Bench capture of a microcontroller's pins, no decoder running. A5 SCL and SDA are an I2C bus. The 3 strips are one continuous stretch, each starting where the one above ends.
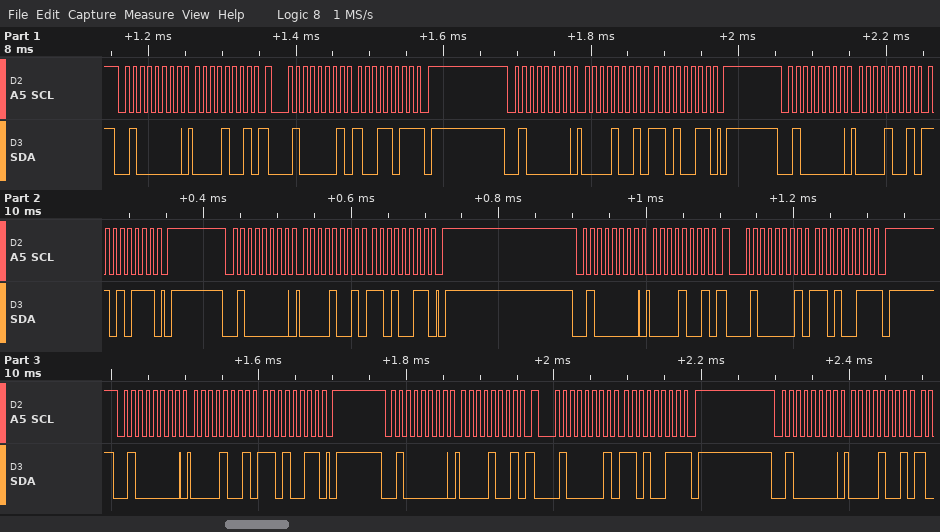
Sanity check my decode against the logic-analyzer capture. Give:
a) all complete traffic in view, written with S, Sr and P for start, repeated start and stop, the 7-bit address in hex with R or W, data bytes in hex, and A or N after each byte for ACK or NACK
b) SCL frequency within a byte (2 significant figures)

S 20W A 09 A Sr 20R A 9B N P S 20W A 09 A D3 A P S 20W A 09 A D7 A P S 20W A 09 A D3 A P S 20W A 09 A Sr 20R A D3 N P S 20W A 09 A D3 A P S 20W A 09 A Sr 20R A D3 N P S 20W A 09 A
100 kHz
